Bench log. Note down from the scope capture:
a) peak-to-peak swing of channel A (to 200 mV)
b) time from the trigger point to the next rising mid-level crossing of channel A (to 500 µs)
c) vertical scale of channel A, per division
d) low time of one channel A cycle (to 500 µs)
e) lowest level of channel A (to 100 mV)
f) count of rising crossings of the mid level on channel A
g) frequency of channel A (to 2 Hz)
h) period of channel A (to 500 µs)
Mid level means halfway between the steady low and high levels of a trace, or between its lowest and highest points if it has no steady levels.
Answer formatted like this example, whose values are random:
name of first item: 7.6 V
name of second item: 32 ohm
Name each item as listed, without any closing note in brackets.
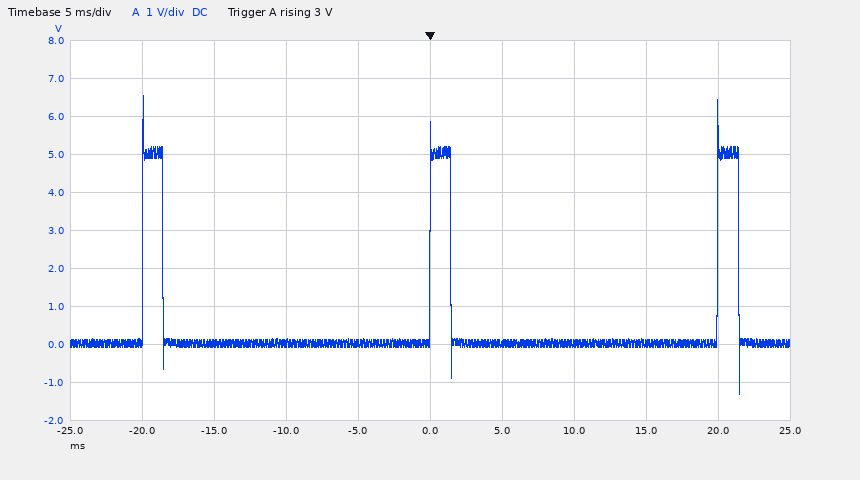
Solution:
peak-to-peak swing of channel A: 7.8 V
time from the trigger point to the next rising mid-level crossing of channel A: 20.0 ms
vertical scale of channel A, per division: 1 V
low time of one channel A cycle: 18.5 ms
lowest level of channel A: -1.3 V
count of rising crossings of the mid level on channel A: 3
frequency of channel A: 50 Hz
period of channel A: 20.0 ms
